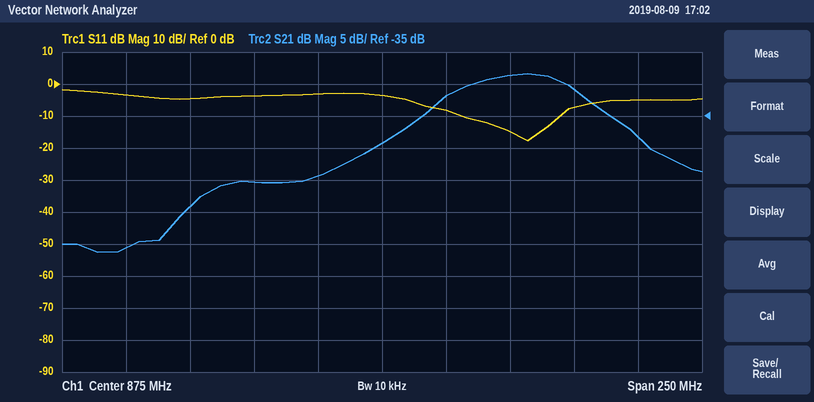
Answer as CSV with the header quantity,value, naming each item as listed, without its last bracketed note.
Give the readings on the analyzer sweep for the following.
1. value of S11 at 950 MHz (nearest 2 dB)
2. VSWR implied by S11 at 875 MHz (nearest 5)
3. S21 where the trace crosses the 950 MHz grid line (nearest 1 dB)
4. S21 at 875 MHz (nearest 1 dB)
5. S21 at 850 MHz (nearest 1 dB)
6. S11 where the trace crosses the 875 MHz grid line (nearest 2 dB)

quantity,value
value of S11 at 950 MHz,-8 dB
VSWR implied by S11 at 875 MHz,5
S21 where the trace crosses the 950 MHz grid line,-31 dB
S21 at 875 MHz,-39 dB
S21 at 850 MHz,-44 dB
S11 where the trace crosses the 875 MHz grid line,-4 dB
